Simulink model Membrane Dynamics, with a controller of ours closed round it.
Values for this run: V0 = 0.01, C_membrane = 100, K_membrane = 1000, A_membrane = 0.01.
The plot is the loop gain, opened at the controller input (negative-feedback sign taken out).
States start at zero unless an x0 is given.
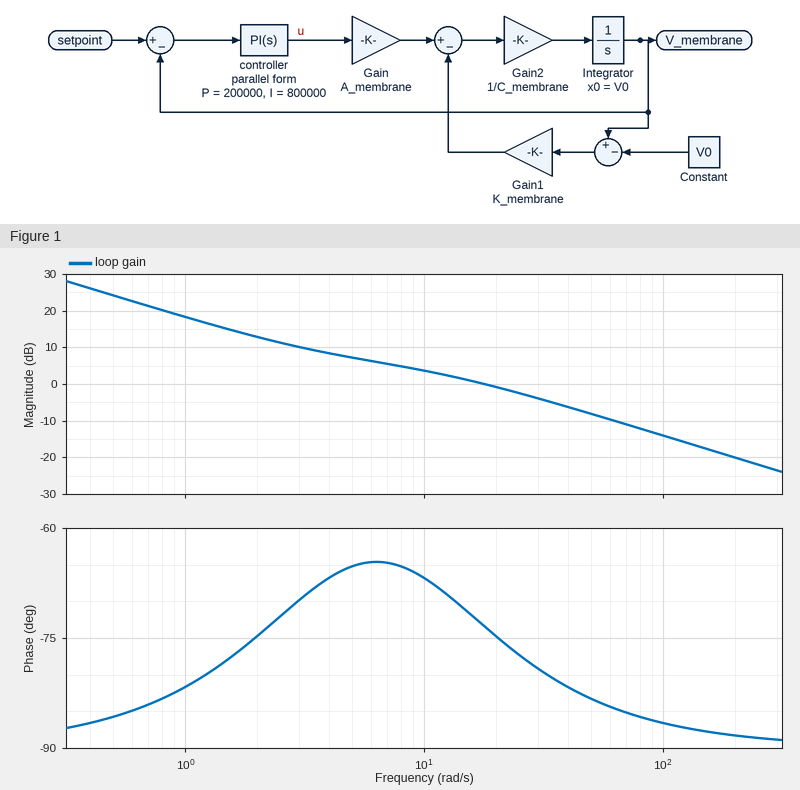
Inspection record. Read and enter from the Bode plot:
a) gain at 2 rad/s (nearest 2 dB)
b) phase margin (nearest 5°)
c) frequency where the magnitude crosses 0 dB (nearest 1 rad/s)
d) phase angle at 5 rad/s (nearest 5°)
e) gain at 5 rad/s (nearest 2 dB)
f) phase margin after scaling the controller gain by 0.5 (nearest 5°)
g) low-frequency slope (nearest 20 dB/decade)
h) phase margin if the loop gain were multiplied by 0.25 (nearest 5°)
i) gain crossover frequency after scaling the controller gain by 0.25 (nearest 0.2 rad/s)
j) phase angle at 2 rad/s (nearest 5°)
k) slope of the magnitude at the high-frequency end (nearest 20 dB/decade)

12 dB
105°
18 rad/s
-65°
8 dB
115°
-20 dB/decade
105°
2.2 rad/s
-75°
-20 dB/decade
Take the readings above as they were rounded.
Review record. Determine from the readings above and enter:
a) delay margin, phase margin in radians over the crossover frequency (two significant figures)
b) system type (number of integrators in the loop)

0.10 s
1
